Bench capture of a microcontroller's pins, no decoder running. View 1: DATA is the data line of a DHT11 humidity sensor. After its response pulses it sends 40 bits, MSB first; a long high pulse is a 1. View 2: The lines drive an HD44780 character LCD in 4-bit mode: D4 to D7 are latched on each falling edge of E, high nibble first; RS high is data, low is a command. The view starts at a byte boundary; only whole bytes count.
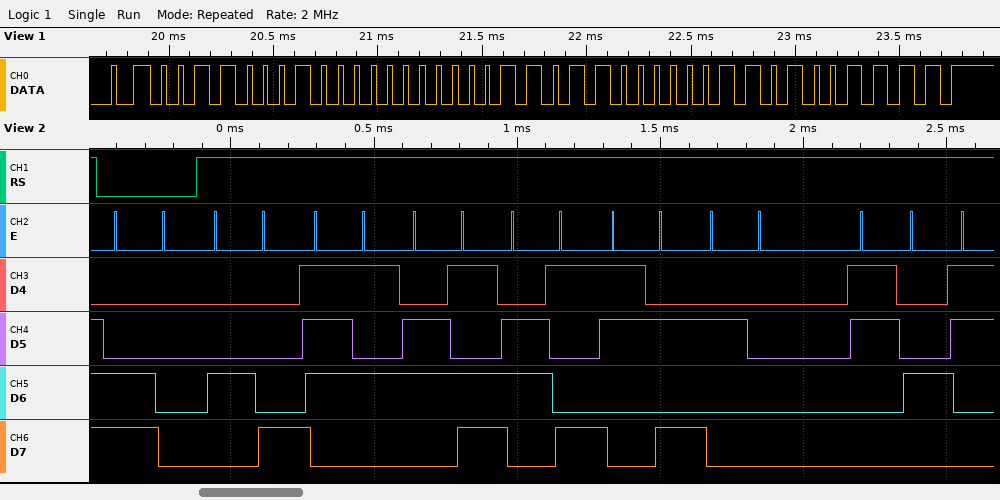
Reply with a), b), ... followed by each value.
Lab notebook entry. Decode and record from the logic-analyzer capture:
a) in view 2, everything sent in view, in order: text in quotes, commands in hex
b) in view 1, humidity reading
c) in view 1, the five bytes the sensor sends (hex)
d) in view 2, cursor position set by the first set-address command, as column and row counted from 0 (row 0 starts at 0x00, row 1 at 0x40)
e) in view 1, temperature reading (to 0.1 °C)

a) 0xC0 "Humi: 4"
b) 49 %
c) 31 00 1B 03 4F
d) column 0, row 1
e) 27.3 °C
